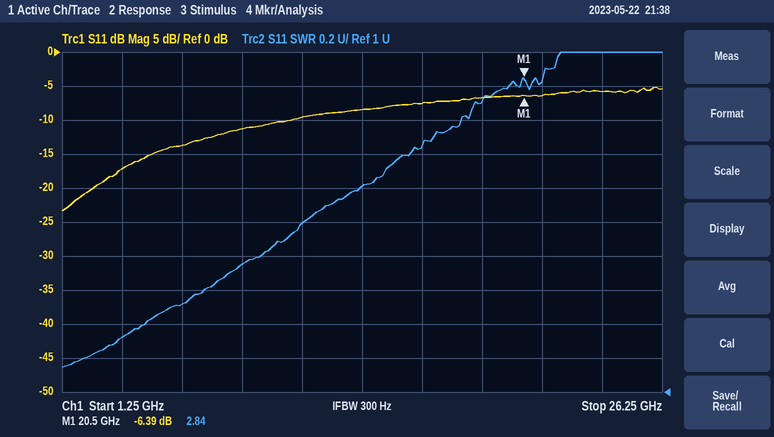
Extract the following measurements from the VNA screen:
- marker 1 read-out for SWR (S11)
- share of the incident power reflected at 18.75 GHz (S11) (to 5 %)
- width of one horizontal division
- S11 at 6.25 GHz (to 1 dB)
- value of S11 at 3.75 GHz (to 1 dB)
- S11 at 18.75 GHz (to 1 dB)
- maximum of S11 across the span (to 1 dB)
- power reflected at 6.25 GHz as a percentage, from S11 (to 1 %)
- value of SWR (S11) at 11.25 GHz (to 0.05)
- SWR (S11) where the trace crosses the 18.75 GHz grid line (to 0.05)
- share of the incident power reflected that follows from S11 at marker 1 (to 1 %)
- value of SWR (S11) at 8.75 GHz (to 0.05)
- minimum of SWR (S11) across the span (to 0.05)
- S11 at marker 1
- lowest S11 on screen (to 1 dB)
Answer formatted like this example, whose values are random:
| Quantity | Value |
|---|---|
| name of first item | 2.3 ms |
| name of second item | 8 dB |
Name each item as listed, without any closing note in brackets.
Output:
| Quantity | Value |
|---|---|
| marker 1 read-out for SWR | 2.84 |
| share of the incident power reflected at 18.75 GHz (S11) | 20 % |
| width of one horizontal division | 2.5 GHz |
| S11 at 6.25 GHz | -14 dB |
| value of S11 at 3.75 GHz | -17 dB |
| S11 at 18.75 GHz | -7 dB |
| maximum of S11 across the span | -5 dB |
| power reflected at 6.25 GHz as a percentage, from S11 | 4 % |
| value of SWR (S11) at 11.25 GHz | 2.00 |
| SWR (S11) where the trace crosses the 18.75 GHz grid line | 2.70 |
| share of the incident power reflected that follows from S11 at marker 1 | 23 % |
| value of SWR (S11) at 8.75 GHz | 1.75 |
| minimum of SWR (S11) across the span | 1.15 |
| S11 at marker 1 | -6.39 dB |
| lowest S11 on screen | -23 dB |
